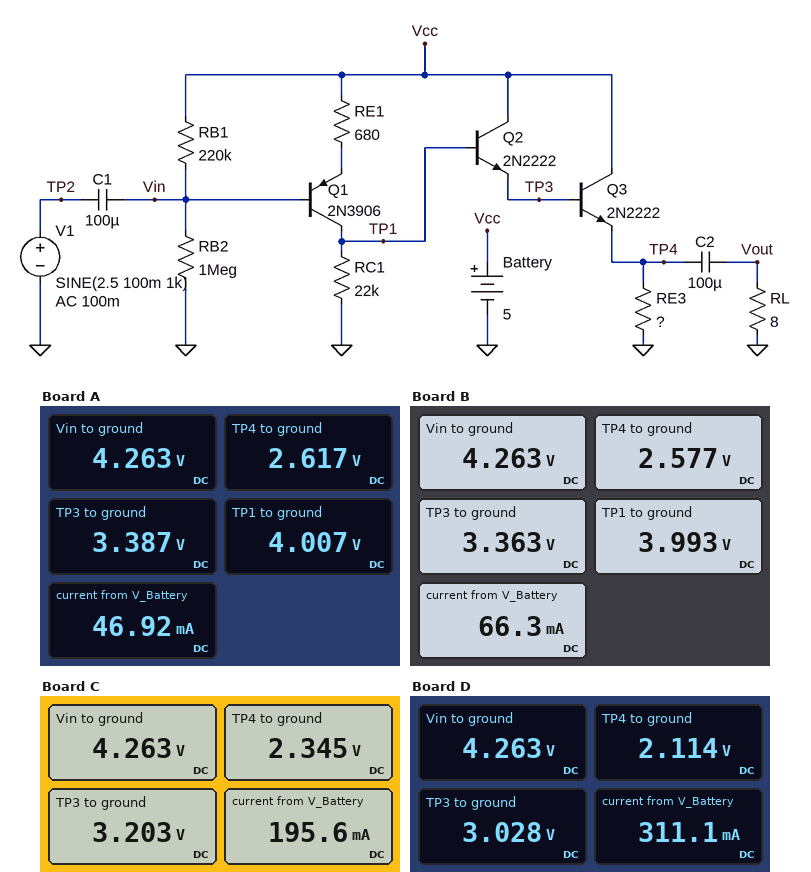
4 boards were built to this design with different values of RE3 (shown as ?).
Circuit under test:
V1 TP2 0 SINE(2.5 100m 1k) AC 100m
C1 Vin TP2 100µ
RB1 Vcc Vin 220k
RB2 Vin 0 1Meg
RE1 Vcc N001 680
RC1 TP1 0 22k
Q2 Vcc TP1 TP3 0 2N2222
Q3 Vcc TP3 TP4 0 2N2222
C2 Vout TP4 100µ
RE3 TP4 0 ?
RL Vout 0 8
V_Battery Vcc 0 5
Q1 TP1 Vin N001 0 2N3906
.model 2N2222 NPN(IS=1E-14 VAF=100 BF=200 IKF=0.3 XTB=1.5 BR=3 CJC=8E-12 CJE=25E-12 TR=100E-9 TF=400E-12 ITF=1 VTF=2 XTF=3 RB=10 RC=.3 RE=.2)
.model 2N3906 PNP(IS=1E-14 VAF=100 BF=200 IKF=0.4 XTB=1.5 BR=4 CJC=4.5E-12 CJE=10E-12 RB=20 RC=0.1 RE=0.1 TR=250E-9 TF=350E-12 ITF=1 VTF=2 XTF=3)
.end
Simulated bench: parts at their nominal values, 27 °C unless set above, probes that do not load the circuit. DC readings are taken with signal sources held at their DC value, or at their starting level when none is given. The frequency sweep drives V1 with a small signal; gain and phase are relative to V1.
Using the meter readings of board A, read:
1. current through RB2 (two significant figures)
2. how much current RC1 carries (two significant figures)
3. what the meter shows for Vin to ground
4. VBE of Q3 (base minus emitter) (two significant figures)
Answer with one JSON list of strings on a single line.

["4.3 µA", "180 µA", "4.263 V", "770 mV"]
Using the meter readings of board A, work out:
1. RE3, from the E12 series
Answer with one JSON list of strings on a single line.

["56 Ω"]
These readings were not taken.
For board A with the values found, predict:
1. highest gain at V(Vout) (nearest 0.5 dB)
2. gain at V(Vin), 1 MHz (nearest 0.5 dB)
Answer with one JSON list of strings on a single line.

["26.0 dB", "0 dB"]
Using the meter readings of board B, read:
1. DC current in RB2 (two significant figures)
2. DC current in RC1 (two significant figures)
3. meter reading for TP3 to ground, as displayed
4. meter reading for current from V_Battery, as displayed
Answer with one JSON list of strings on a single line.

["4.3 µA", "180 µA", "3.363 V", "66.3 mA"]
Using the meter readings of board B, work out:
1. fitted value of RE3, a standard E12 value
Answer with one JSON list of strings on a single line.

["39 Ω"]
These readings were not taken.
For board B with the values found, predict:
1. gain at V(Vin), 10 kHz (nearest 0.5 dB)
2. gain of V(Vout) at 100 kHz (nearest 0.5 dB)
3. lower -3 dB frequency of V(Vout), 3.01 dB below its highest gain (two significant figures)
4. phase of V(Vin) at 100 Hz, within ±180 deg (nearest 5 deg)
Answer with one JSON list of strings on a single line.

["0 dB", "26.0 dB", "160 Hz", "0 deg"]
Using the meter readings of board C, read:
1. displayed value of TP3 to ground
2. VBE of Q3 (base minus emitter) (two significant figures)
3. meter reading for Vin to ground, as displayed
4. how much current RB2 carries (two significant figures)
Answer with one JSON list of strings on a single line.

["3.203 V", "860 mV", "4.263 V", "4.3 µA"]
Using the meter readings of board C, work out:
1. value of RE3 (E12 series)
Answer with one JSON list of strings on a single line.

["12 Ω"]
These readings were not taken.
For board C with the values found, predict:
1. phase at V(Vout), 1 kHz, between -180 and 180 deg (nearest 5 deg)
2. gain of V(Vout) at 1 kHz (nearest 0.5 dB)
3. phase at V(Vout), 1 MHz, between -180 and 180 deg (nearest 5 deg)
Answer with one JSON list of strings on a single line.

["-170 deg", "25.5 dB", "120 deg"]
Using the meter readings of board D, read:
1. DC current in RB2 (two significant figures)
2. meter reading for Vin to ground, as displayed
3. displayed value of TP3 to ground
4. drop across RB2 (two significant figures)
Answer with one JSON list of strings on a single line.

["4.3 µA", "4.263 V", "3.028 V", "4.3 V"]
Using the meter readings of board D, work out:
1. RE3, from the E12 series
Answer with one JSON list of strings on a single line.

["6.8 Ω"]
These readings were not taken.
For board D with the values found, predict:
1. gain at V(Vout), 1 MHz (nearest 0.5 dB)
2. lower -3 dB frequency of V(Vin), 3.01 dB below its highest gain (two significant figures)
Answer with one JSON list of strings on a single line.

["20.5 dB", "19 mHz"]
